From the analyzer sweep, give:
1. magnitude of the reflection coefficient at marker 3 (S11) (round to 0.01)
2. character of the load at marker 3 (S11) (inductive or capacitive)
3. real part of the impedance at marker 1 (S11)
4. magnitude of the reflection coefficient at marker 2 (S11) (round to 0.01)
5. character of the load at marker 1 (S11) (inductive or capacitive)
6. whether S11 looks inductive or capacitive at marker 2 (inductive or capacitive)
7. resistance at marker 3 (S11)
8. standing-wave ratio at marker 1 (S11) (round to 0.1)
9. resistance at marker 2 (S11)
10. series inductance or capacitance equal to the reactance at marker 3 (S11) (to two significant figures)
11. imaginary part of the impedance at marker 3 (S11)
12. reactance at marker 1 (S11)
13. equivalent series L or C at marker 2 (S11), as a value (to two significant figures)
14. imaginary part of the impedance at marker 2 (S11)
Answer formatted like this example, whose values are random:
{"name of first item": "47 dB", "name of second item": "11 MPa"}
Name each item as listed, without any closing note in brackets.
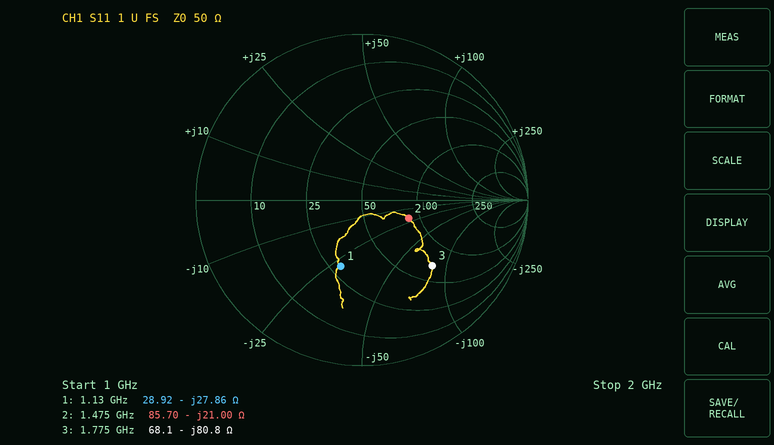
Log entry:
{"magnitude of the reflection coefficient at marker 3 (S11)": "0.58", "character of the load at marker 3 (S11)": "capacitive", "real part of the impedance at marker 1": "28.92 Ω", "magnitude of the reflection coefficient at marker 2 (S11)": "0.30", "character of the load at marker 1 (S11)": "capacitive", "whether S11 looks inductive or capacitive at marker 2": "capacitive", "resistance at marker 3": "68.1 Ω", "standing-wave ratio at marker 1 (S11)": "2.4", "resistance at marker 2": "85.70 Ω", "series inductance or capacitance equal to the reactance at marker 3 (S11)": "1.1 pF", "imaginary part of the impedance at marker 3": "-80.8 Ω", "reactance at marker 1": "-27.86 Ω", "equivalent series L or C at marker 2 (S11), as a value": "5.1 pF", "imaginary part of the impedance at marker 2": "-21.00 Ω"}
